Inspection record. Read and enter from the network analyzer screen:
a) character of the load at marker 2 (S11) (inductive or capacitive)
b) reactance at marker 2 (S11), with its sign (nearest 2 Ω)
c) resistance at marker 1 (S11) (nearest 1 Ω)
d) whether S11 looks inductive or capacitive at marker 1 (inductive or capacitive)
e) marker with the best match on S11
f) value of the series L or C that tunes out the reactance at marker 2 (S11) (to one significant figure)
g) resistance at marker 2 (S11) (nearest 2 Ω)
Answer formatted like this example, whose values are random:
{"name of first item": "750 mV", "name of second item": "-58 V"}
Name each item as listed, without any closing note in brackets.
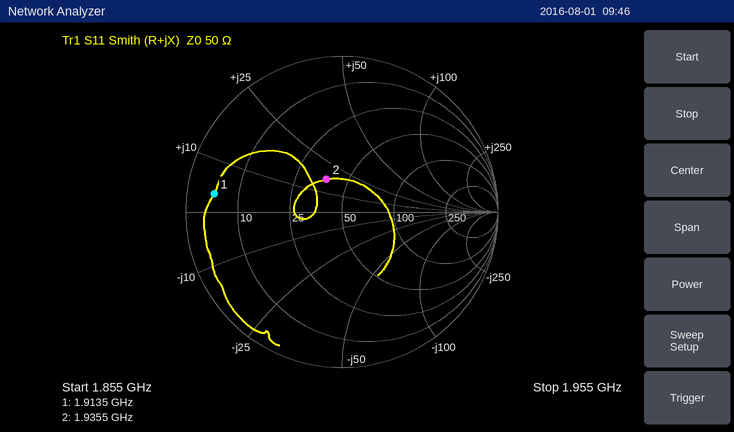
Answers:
{"character of the load at marker 2 (S11)": "inductive", "reactance at marker 2 (S11), with its sign": "+16 Ω", "resistance at marker 1 (S11)": "5 Ω", "whether S11 looks inductive or capacitive at marker 1": "inductive", "marker with the best match on S11": "marker 2", "value of the series L or C that tunes out the reactance at marker 2 (S11)": "5 pF", "resistance at marker 2 (S11)": "38 Ω"}
